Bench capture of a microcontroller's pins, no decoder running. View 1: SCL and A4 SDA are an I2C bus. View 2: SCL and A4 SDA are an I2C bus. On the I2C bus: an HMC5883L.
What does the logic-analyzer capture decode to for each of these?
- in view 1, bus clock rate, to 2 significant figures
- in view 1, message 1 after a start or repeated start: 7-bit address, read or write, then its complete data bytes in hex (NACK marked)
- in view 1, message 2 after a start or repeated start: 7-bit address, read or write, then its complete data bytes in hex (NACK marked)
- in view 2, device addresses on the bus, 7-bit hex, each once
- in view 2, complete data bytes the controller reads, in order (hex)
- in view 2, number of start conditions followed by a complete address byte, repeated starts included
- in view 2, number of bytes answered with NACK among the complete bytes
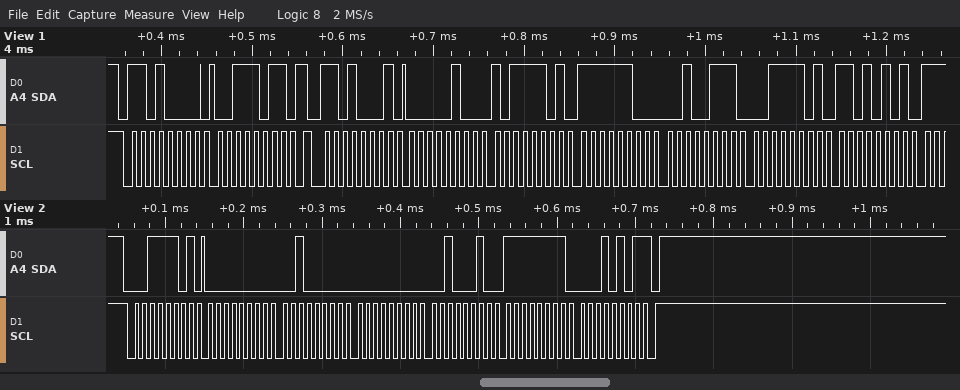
100 kHz
0x68 write: 3B
0x68 read: 04 BD FC 27 3D D5
0x1E
00 20 00 22 FF 15
1
1
